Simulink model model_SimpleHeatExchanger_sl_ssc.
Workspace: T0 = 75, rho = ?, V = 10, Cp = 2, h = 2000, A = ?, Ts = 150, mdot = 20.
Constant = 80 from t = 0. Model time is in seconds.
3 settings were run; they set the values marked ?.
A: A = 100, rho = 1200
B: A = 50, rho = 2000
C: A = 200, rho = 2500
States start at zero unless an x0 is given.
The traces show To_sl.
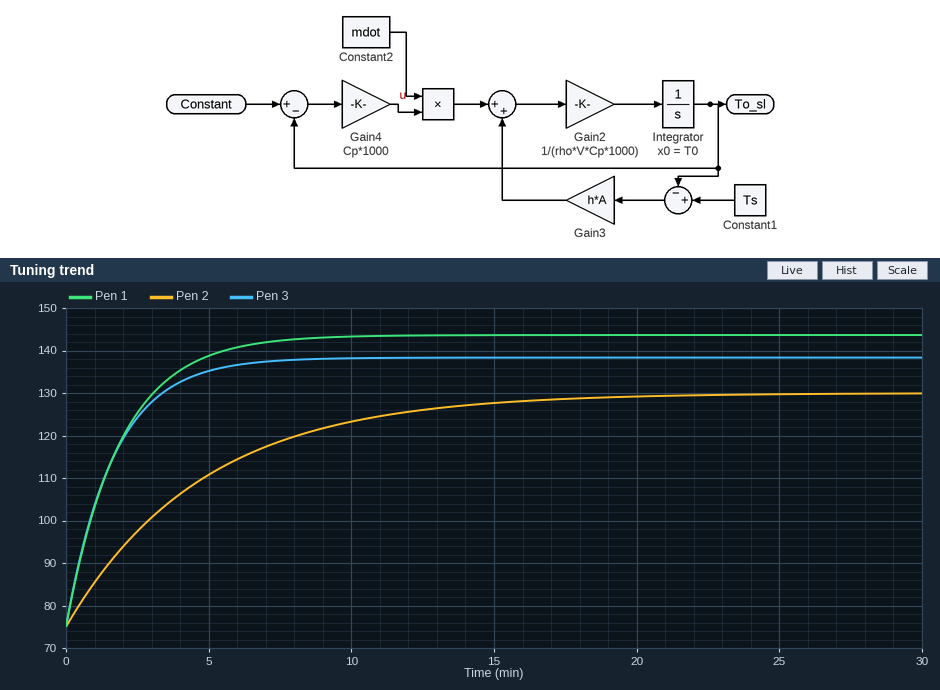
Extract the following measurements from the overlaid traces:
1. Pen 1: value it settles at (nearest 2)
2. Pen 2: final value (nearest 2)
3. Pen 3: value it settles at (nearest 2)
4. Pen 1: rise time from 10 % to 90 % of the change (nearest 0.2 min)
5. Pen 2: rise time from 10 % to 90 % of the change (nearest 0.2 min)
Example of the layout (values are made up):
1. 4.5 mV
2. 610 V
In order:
1. 144
2. 130
3. 138
4. 4.2 min
5. 10.4 min
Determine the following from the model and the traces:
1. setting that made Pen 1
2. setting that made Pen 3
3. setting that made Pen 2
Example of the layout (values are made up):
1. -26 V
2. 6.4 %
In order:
1. C
2. A
3. B
